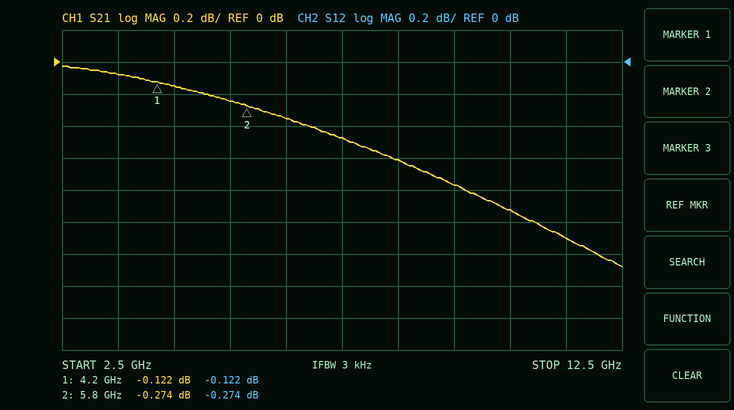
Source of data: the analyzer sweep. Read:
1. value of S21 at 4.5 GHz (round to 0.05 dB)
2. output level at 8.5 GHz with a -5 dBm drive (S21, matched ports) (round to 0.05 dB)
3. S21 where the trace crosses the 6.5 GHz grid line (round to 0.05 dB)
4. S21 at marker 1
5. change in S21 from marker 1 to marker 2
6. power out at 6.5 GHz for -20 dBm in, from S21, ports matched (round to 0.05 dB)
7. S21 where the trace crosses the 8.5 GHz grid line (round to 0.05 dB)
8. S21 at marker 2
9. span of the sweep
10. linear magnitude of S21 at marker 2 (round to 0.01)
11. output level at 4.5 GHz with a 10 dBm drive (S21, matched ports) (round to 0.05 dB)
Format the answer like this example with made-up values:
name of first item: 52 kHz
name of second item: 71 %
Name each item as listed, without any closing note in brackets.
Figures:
value of S21 at 4.5 GHz: -0.15 dB
output level at 8.5 GHz with a -5 dBm drive (S21, matched ports): -5.60 dBm
S21 where the trace crosses the 6.5 GHz grid line: -0.35 dB
S21 at marker 1: -0.122 dB
change in S21 from marker 1 to marker 2: -0.152 dB
power out at 6.5 GHz for -20 dBm in, from S21, ports matched: -20.35 dBm
S21 where the trace crosses the 8.5 GHz grid line: -0.60 dB
S21 at marker 2: -0.274 dB
span of the sweep: 10 GHz
linear magnitude of S21 at marker 2: 0.97
output level at 4.5 GHz with a 10 dBm drive (S21, matched ports): 9.85 dBm
